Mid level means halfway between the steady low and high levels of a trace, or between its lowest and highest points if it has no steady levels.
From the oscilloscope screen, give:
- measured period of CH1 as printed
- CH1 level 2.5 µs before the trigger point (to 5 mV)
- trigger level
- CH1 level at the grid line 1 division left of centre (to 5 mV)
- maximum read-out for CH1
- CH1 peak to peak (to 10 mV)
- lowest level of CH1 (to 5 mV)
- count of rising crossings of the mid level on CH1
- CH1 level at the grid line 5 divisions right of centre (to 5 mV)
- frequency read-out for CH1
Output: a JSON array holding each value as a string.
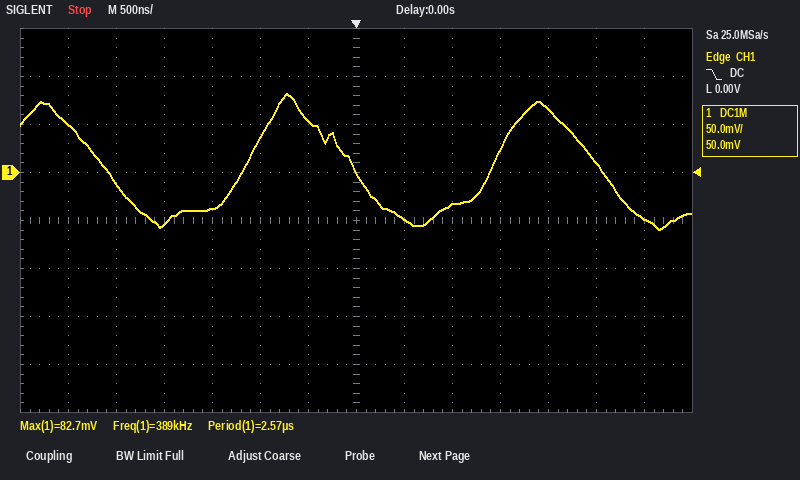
["2.57 µs", "-10 mV", "0.00 V", "55 mV", "82.7 mV", "140 mV", "-60 mV", "2", "10 mV", "389 kHz"]
